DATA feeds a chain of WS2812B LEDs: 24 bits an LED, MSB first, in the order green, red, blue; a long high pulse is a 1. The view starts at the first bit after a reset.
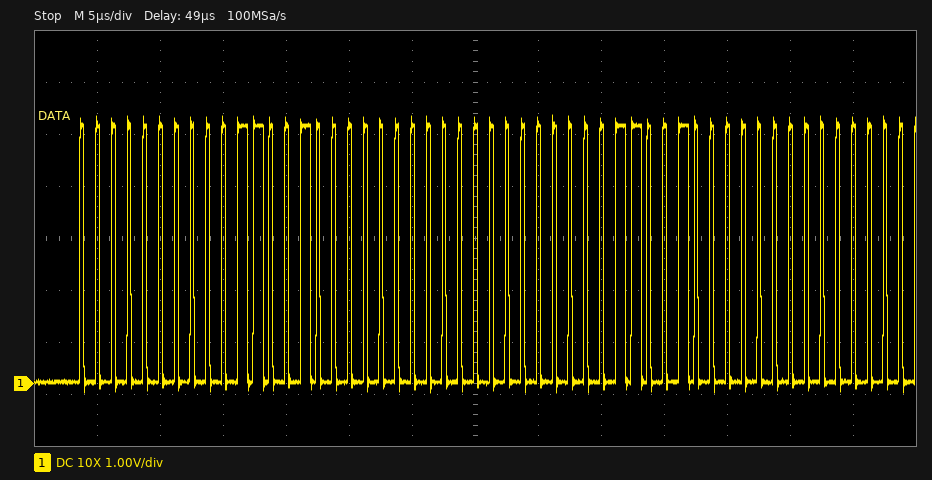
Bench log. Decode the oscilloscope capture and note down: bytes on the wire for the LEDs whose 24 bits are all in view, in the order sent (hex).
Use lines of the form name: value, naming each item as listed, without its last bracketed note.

bytes on the wire for the LEDs whose 24 bits are all in view, in the order sent: 00 32 00 00 32 00
